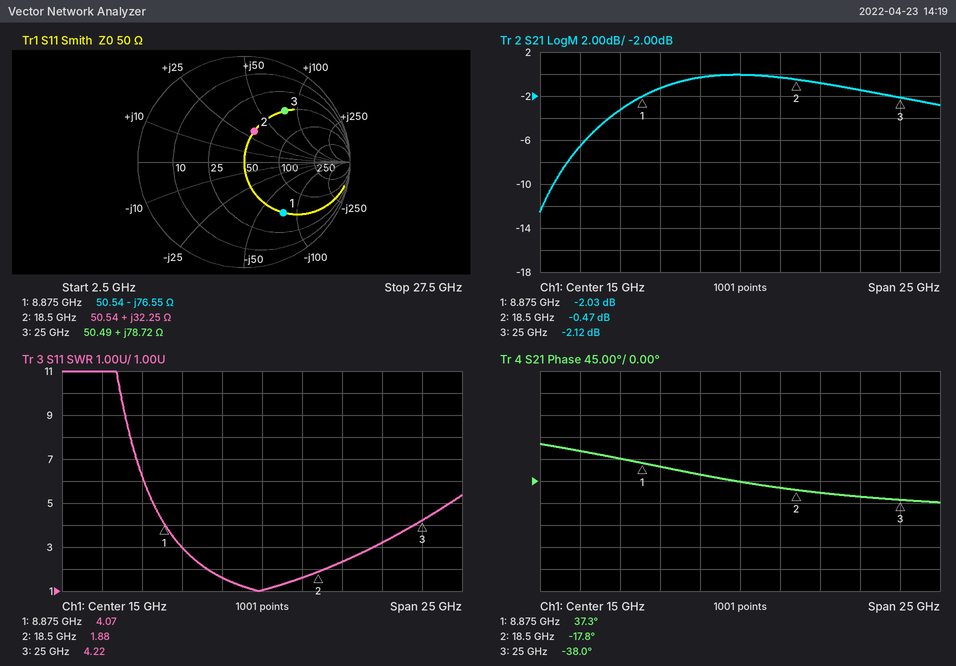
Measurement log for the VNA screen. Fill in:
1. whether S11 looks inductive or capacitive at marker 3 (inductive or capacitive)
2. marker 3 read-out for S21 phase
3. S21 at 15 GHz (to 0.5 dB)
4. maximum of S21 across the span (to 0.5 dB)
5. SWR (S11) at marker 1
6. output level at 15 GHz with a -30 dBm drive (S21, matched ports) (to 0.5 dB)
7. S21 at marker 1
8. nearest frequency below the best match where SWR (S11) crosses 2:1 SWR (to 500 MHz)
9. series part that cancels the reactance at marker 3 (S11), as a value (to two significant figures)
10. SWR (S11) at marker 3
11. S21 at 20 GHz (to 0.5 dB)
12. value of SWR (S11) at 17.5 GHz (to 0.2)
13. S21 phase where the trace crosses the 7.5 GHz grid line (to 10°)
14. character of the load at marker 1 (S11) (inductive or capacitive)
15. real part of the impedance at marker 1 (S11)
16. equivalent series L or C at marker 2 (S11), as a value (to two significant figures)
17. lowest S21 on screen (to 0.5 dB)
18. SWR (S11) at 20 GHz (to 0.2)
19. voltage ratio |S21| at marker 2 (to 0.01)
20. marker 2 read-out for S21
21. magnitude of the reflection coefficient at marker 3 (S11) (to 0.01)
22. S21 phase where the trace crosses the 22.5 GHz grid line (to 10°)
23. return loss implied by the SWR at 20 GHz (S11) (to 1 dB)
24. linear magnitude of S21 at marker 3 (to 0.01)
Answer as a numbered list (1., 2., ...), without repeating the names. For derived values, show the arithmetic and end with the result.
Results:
1. inductive
2. -38.0°
3. 0.0 dB
4. 0.0 dB
5. 4.07
6. -30 dBm + (0.0 dB) = -30.0 dBm
7. -2.03 dB
8. 11.5 GHz
9. C = 1/(2π × 25 GHz × 78.72 Ω) ≈ 81 fF
10. 4.22
11. -1.0 dB
12. 1.6
13. 50°
14. capacitive
15. 50.54 Ω
16. L = 32.25 Ω/(2π × 18.5 GHz) ≈ 277 pH, so 280 pH to two significant figures
17. -12.5 dB
18. 2.4
19. 10^(-0.47/20) ≈ 0.95
20. -0.47 dB
21. 0.62
22. -30°
23. −20 log10((2.4 − 1)/(2.4 + 1)) ≈ 8 dB
24. 10^(-2.12/20) ≈ 0.78
